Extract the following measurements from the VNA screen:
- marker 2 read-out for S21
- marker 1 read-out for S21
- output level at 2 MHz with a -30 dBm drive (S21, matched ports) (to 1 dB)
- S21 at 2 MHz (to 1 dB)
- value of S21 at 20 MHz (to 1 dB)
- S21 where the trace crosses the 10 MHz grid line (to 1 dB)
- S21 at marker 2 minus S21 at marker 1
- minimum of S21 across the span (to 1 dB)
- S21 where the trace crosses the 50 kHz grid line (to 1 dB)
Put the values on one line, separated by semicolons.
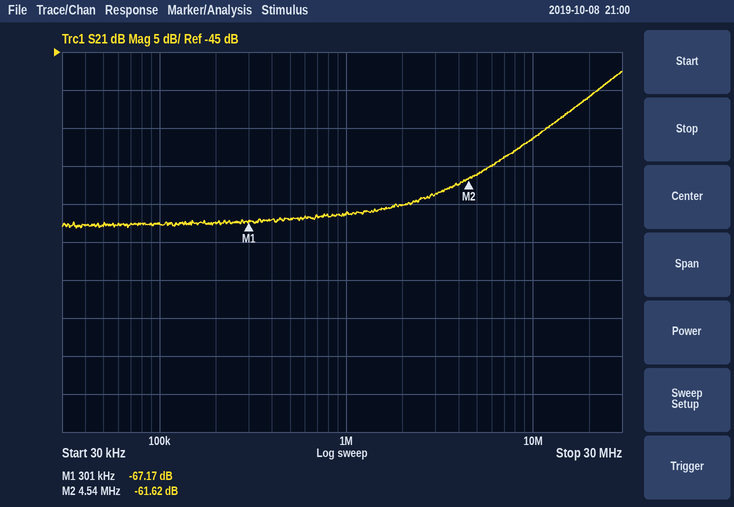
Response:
-61.62 dB; -67.17 dB; -95 dBm; -65 dB; -51 dB; -56 dB; 5.55 dB; -68 dB; -68 dB
